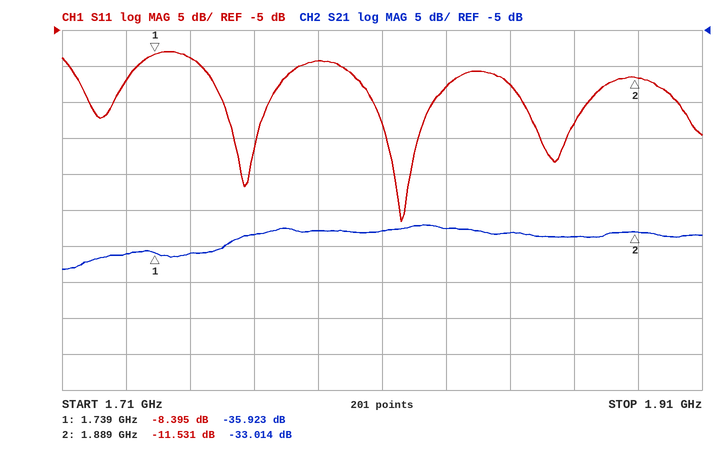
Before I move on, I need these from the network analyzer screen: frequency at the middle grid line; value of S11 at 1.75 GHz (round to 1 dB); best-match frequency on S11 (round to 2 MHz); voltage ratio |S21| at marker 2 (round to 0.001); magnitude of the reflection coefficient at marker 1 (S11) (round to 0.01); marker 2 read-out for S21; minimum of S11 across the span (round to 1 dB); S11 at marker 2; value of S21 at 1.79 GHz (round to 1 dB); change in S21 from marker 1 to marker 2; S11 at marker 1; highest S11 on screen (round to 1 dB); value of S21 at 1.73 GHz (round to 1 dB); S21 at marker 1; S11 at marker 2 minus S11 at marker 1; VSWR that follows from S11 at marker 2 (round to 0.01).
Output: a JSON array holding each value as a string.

["1.81 GHz", "-9 dB", "1.816 GHz", "0.022", "0.38", "-33.014 dB", "-32 dB", "-11.531 dB", "-33 dB", "2.909 dB", "-8.395 dB", "-8 dB", "-36 dB", "-35.923 dB", "-3.136 dB", "1.72"]
